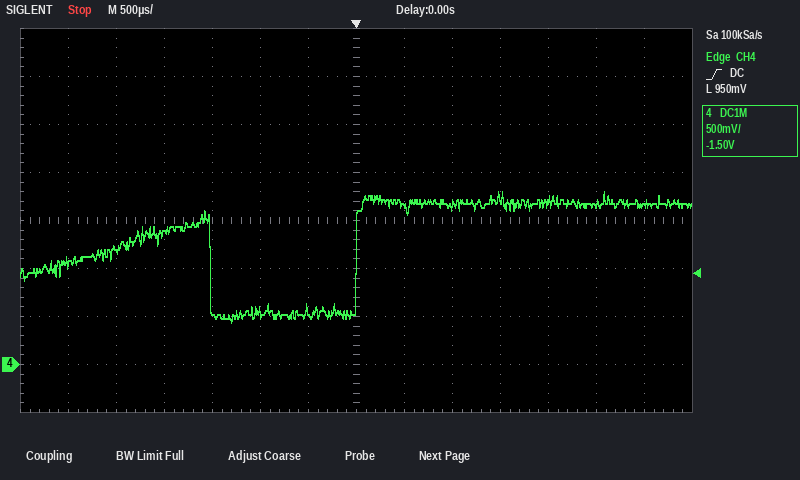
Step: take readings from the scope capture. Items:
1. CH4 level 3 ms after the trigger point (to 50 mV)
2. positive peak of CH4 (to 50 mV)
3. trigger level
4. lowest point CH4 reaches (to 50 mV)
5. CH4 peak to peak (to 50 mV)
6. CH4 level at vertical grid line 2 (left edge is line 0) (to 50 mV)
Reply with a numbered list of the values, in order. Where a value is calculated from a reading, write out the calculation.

1. 1.65 V
2. 1.80 V
3. 950 mV
4. 450 mV
5. 1.80 V − (450 mV) = 1.35 V
6. 1.20 V
